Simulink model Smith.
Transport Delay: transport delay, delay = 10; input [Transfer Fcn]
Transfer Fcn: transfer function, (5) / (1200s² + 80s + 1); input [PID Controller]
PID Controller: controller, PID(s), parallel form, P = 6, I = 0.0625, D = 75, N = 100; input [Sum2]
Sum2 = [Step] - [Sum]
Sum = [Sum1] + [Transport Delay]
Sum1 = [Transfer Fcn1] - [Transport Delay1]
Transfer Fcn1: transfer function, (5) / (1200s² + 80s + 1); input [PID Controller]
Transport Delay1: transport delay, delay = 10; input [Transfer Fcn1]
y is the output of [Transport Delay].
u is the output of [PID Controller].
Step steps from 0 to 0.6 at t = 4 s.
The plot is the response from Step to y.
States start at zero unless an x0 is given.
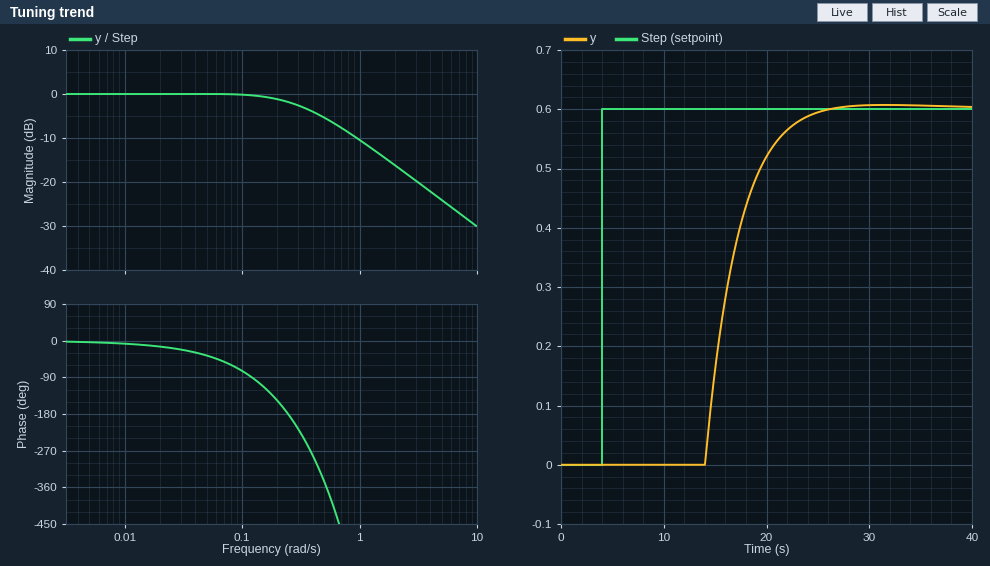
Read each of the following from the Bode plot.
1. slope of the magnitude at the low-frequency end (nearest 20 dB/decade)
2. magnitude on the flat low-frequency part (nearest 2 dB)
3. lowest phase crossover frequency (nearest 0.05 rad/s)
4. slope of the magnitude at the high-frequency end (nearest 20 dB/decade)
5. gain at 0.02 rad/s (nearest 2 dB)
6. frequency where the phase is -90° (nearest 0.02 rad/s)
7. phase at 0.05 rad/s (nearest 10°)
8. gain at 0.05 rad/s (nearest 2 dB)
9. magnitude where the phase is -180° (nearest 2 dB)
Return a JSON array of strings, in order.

["0 dB/decade", "0 dB", "0.25 rad/s", "-20 dB/decade", "0 dB", "0.12 rad/s", "-40°", "0 dB", "-2 dB"]
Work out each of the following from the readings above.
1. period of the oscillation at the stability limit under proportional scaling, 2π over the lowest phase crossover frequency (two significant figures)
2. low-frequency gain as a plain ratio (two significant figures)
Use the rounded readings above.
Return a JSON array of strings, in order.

["25 s", "1.0"]
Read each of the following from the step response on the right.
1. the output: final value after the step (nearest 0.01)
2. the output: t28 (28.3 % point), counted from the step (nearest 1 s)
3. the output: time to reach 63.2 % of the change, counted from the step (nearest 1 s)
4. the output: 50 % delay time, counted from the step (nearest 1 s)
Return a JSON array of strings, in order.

["0.60", "11 s", "13 s", "12 s"]
